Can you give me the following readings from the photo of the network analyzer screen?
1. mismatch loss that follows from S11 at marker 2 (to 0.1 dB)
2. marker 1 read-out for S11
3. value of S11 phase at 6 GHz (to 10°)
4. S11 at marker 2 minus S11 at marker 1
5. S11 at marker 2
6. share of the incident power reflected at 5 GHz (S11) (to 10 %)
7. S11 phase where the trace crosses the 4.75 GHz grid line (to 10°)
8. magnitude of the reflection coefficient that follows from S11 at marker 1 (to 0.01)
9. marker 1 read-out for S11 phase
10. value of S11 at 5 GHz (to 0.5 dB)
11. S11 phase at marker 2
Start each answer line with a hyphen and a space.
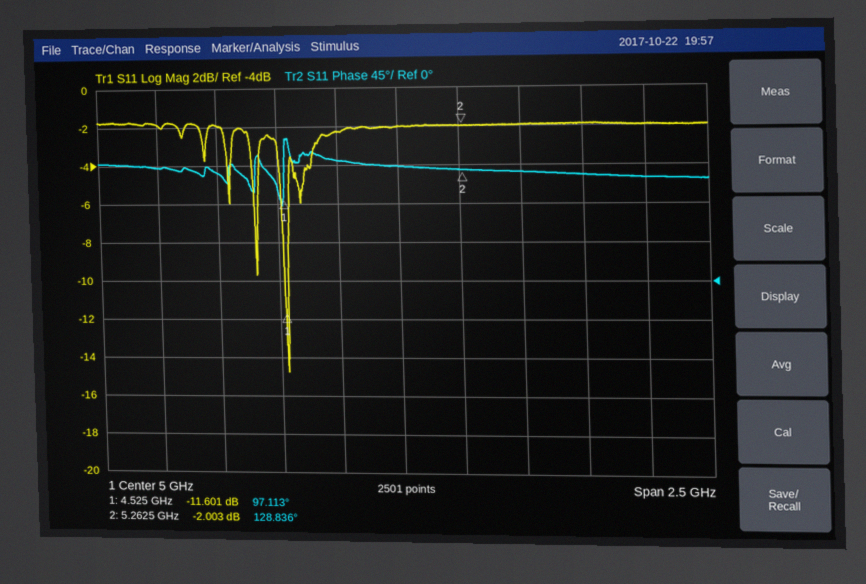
- 4.3 dB
- -11.601 dB
- 120°
- 9.598 dB
- -2.003 dB
- 60 %
- 140°
- 0.26
- 97.113°
- -2.0 dB
- 128.836°
